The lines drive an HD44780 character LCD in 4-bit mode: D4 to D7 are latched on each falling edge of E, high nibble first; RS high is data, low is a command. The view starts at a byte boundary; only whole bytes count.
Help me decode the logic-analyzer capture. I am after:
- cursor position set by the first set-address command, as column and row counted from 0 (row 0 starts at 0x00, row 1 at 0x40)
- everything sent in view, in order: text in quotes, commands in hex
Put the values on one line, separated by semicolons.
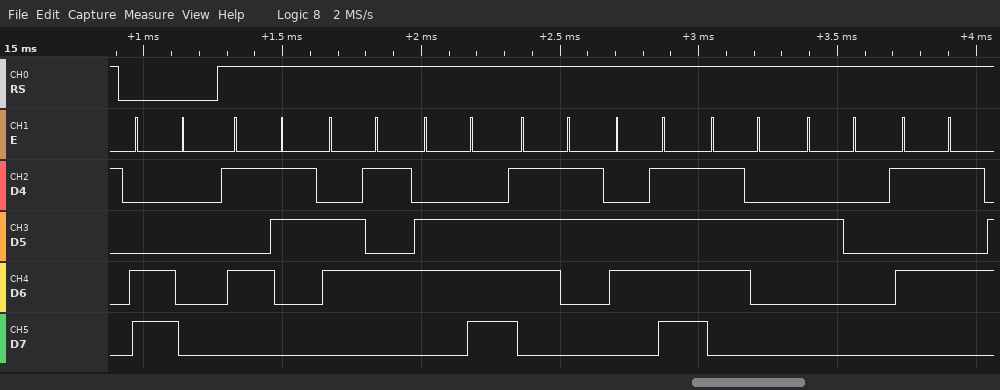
column 0, row 1; 0xC0 "Sensor U"
